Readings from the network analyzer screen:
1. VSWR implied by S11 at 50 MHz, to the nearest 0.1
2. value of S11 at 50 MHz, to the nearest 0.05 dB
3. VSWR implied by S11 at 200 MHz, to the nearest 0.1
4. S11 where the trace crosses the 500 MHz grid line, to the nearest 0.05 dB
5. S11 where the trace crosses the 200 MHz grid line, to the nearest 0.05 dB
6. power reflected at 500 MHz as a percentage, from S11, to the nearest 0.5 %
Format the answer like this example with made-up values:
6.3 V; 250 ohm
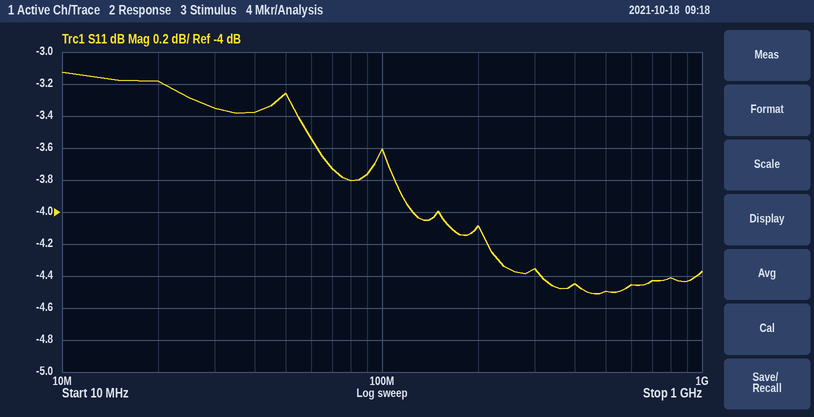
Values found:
5.4; -3.25 dB; 4.3; -4.50 dB; -4.10 dB; 35.5 %
